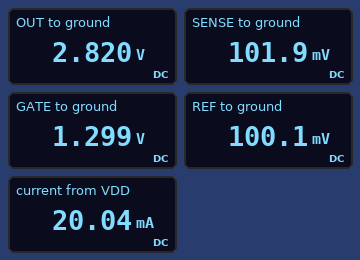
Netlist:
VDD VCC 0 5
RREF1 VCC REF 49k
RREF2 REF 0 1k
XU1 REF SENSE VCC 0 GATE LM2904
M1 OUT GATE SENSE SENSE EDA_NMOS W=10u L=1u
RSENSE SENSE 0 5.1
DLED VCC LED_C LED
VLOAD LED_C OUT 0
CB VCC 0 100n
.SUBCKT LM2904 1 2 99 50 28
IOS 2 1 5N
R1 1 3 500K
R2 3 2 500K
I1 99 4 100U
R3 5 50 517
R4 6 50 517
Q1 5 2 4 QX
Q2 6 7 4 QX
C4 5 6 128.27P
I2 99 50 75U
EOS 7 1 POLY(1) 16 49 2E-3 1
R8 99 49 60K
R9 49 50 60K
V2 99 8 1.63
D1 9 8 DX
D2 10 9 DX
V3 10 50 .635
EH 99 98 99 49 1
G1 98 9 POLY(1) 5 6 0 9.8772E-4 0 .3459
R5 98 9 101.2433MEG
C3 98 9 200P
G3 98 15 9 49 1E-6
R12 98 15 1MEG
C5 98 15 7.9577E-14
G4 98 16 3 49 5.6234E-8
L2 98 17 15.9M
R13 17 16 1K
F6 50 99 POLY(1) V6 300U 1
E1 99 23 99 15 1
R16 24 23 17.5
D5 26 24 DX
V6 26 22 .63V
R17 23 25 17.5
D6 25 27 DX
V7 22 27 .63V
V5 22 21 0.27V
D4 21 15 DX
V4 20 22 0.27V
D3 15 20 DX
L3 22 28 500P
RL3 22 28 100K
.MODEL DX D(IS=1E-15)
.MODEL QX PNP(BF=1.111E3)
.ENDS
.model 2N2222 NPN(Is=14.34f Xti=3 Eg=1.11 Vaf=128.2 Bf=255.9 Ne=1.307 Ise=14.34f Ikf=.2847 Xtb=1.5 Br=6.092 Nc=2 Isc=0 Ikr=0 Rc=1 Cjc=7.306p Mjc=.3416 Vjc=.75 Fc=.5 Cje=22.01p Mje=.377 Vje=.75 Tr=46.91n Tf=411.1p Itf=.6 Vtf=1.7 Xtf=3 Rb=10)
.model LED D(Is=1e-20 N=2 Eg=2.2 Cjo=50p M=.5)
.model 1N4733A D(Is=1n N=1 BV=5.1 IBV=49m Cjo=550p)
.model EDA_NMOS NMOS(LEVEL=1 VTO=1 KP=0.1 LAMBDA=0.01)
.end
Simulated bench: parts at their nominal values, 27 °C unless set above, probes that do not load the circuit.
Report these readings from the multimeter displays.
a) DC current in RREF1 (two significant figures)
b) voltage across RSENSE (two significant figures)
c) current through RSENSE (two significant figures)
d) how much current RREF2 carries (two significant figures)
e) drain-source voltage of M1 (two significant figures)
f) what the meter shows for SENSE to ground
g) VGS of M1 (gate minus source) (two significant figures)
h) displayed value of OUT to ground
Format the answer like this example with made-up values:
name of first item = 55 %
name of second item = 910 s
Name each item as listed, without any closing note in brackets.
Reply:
DC current in RREF1 = 100 µA
voltage across RSENSE = 100 mV
current through RSENSE = 20 mA
how much current RREF2 carries = 100 µA
drain-source voltage of M1 = 2.7 V
what the meter shows for SENSE to ground = 101.9 mV
VGS of M1 (gate minus source) = 1.2 V
displayed value of OUT to ground = 2.820 V
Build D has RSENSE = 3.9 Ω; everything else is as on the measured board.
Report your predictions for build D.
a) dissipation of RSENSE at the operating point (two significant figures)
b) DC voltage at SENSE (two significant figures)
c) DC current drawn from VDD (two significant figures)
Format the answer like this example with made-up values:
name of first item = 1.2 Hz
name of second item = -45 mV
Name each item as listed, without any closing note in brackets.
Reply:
dissipation of RSENSE at the operating point = 2.7 mW
DC voltage at SENSE = 100 mV
DC current drawn from VDD = 26 mA
